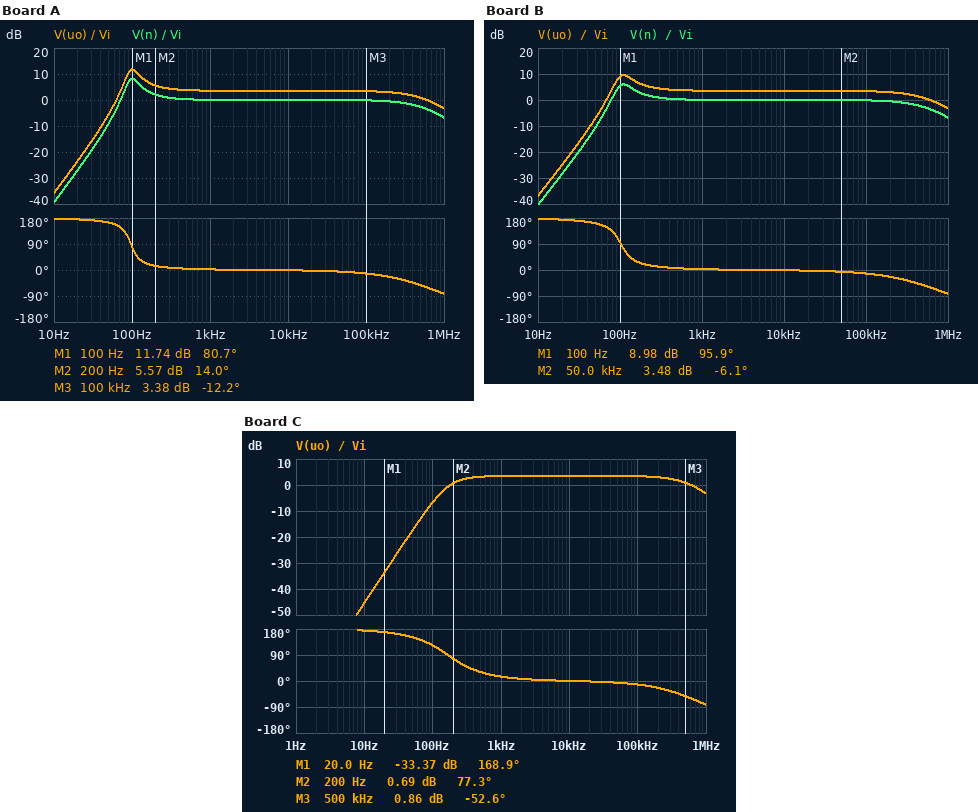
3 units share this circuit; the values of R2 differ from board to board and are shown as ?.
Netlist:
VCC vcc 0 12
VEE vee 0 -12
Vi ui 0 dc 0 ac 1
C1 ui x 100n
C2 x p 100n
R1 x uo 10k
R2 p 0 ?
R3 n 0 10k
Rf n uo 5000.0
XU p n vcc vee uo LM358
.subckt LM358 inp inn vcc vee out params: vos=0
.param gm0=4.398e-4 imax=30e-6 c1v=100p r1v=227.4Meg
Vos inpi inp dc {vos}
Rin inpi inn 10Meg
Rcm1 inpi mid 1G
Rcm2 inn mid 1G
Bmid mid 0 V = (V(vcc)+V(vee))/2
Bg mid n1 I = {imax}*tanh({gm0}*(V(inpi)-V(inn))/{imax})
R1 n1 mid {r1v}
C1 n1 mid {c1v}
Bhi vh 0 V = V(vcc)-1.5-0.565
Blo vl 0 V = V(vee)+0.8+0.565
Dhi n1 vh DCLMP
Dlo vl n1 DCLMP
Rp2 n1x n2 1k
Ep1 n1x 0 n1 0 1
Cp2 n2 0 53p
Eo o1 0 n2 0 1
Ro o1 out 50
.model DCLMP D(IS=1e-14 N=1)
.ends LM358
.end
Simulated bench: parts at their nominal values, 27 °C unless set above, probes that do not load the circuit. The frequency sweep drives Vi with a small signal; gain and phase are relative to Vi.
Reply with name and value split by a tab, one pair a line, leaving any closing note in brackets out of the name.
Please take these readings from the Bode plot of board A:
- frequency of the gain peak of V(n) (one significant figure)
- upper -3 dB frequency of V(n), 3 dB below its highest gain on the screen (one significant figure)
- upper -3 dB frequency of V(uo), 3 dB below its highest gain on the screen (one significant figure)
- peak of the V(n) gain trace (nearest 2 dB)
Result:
frequency of the gain peak of V(n)	100 Hz
upper -3 dB frequency of V(n), 3 dB below its highest gain on the screen	100 Hz
upper -3 dB frequency of V(uo), 3 dB below its highest gain on the screen	100 Hz
peak of the V(n) gain trace	8 dB
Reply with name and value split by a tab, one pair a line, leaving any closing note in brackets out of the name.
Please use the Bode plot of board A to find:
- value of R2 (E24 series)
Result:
value of R2	27 kΩ
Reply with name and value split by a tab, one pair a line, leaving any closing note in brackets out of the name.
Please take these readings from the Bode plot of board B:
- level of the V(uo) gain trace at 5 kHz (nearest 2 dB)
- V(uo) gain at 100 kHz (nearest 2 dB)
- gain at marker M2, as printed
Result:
level of the V(uo) gain trace at 5 kHz	4 dB
V(uo) gain at 100 kHz	4 dB
gain at marker M2, as printed	3.48 dB
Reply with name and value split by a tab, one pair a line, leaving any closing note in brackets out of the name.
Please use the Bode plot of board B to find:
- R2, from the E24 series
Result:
R2, from the E24 series	24 kΩ
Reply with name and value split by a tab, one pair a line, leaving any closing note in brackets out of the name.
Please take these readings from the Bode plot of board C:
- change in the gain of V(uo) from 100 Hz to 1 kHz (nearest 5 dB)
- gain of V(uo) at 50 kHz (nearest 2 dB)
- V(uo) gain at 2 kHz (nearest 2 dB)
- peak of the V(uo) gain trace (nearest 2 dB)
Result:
change in the gain of V(uo) from 100 Hz to 1 kHz	10 dB
gain of V(uo) at 50 kHz	4 dB
V(uo) gain at 2 kHz	4 dB
peak of the V(uo) gain trace	4 dB
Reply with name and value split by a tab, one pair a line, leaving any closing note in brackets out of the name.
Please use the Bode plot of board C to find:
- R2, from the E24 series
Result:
R2, from the E24 series	9.1 kΩ
